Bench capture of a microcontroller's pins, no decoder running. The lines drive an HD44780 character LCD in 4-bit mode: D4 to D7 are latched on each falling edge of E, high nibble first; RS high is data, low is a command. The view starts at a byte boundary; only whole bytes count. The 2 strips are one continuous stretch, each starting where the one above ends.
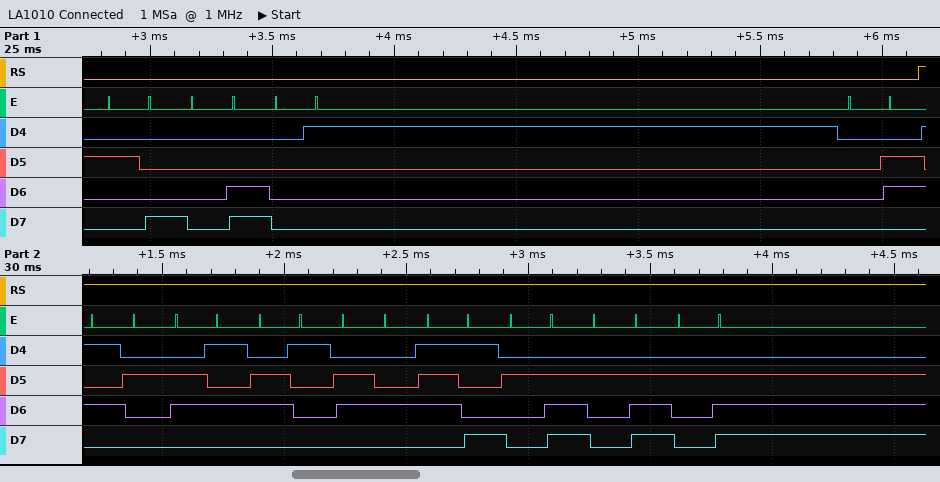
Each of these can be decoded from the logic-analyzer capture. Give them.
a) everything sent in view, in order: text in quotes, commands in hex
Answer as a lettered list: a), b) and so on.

a) 0x28 0x0C 0x01 0x06 "Ready..."
